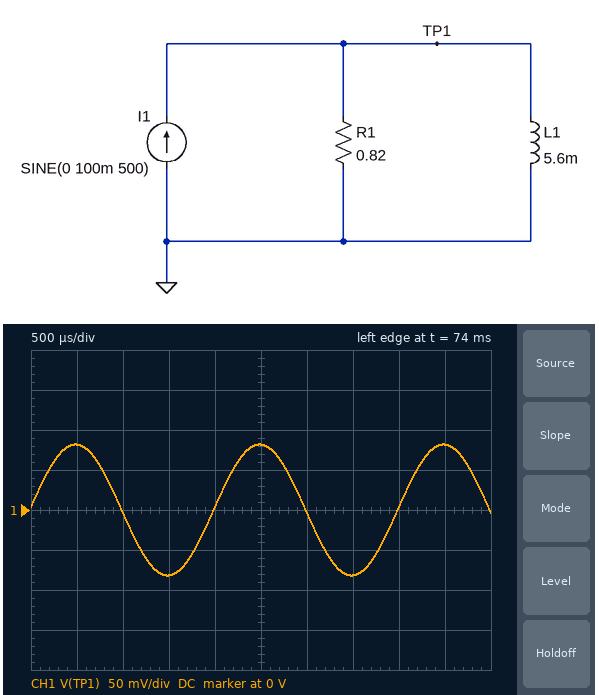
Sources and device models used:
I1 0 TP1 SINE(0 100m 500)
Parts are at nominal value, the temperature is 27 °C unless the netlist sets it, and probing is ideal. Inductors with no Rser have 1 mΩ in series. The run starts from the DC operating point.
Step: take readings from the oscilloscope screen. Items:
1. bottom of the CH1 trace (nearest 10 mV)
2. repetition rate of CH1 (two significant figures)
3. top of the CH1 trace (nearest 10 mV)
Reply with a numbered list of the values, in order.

1. -80 mV
2. 500 Hz
3. 80 mV
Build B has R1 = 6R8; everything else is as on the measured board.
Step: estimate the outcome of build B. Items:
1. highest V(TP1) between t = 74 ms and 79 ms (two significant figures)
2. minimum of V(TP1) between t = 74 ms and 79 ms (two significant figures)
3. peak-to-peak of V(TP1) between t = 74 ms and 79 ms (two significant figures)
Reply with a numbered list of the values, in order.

1. 630 mV
2. -630 mV
3. 1.3 V
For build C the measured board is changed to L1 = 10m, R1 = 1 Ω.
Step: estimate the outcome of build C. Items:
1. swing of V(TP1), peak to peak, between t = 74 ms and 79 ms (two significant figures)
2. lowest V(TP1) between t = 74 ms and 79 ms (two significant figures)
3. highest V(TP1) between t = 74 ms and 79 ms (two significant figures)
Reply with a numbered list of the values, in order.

1. 200 mV
2. -100 mV
3. 100 mV
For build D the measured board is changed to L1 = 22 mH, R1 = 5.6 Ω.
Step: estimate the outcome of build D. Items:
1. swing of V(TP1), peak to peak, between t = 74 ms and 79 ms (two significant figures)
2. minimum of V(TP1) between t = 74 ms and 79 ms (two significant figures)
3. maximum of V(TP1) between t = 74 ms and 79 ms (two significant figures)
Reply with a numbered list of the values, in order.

1. 1.1 V
2. -560 mV
3. 560 mV
